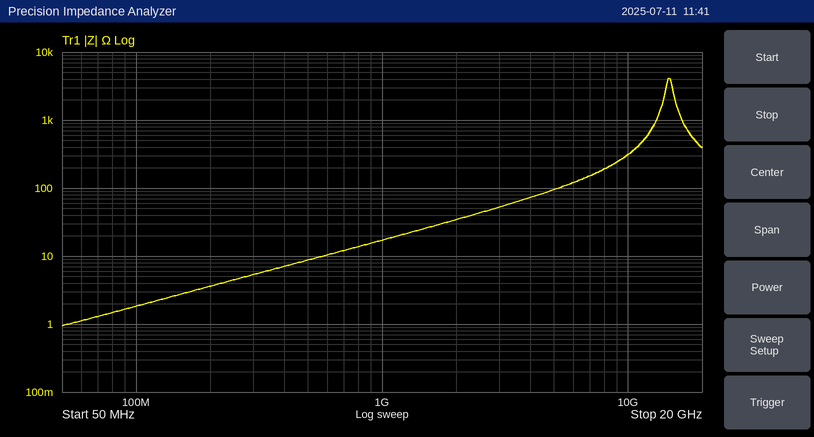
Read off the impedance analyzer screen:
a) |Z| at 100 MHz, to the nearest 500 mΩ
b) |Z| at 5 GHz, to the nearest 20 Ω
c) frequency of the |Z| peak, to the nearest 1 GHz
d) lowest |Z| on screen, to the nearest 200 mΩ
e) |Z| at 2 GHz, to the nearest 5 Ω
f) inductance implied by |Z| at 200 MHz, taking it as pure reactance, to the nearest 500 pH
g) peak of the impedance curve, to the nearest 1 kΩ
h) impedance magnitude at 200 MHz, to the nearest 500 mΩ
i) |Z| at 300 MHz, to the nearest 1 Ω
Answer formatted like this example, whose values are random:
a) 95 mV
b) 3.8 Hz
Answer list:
a) 2.0 Ω
b) 100 Ω
c) 15 GHz
d) 1.0 Ω
e) 35 Ω
f) 3.0 nH
g) 4 kΩ
h) 3.5 Ω
i) 5 Ω
